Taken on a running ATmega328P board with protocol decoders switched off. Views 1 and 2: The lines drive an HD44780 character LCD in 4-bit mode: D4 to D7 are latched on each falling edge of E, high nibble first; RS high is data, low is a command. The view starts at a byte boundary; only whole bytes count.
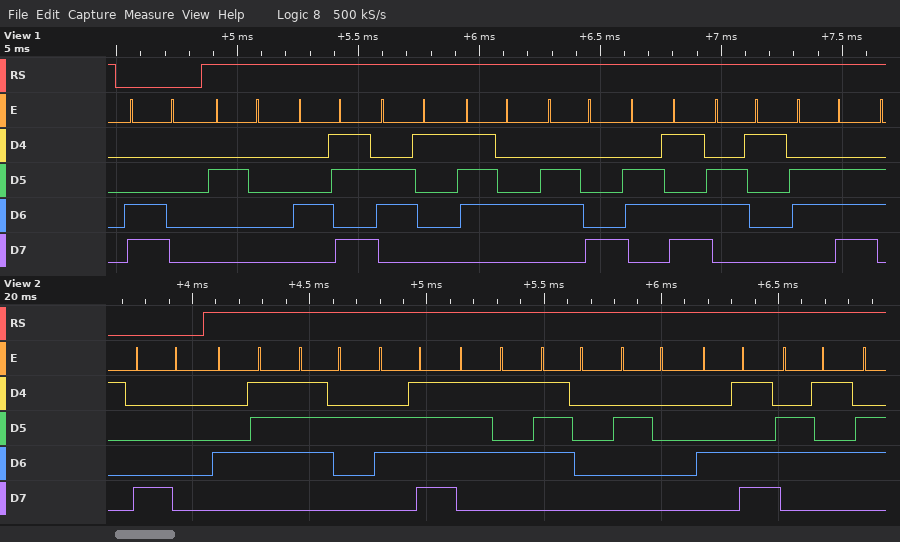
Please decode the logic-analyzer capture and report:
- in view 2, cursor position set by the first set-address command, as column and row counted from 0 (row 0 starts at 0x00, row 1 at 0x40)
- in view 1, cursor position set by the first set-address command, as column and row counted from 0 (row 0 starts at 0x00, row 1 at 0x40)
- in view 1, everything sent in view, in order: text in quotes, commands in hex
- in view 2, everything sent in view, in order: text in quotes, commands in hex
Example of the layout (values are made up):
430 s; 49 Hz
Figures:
column 0, row 0; column 0, row 1; 0xC0 " Kathman"; 0x80 "Group Me"
